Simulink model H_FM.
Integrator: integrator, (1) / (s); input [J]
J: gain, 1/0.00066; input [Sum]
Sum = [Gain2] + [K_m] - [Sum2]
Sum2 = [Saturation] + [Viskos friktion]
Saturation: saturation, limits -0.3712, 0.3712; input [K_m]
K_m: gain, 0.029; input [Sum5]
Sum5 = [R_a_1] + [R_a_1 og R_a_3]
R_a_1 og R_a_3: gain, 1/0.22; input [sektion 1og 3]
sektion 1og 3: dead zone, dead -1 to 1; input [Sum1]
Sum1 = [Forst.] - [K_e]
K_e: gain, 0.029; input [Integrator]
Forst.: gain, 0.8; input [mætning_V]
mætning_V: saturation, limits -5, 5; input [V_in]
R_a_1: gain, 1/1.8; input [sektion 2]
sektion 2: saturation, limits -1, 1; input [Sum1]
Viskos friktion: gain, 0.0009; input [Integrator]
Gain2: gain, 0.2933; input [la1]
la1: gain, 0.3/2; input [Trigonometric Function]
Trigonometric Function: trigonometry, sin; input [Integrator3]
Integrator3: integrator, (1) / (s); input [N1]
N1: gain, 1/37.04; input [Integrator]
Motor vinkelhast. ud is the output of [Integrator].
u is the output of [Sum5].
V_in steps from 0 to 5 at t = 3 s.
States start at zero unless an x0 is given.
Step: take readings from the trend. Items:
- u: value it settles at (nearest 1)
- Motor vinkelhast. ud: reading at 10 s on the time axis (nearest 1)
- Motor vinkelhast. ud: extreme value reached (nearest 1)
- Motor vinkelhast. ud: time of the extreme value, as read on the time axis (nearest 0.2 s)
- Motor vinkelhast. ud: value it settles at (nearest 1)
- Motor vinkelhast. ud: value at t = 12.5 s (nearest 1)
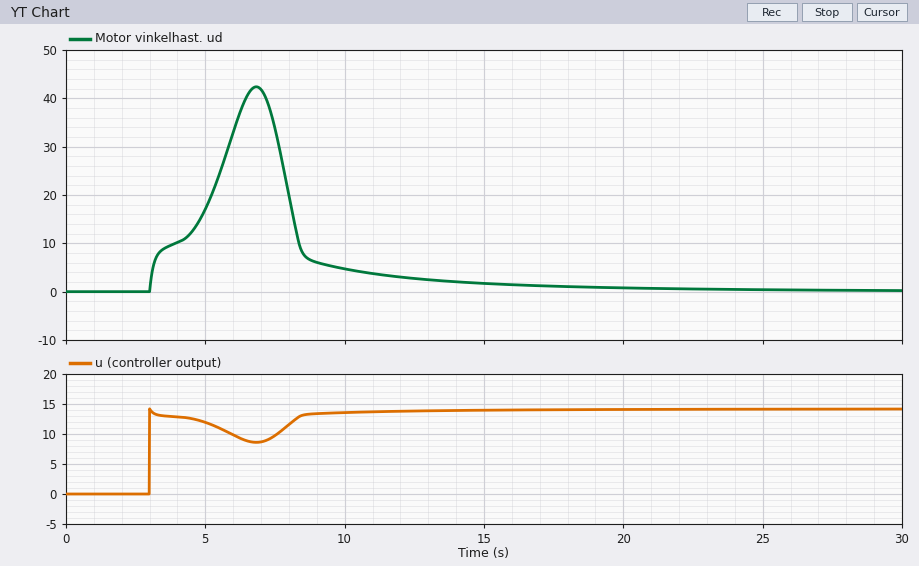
14
5
42
6.8 s
0
3
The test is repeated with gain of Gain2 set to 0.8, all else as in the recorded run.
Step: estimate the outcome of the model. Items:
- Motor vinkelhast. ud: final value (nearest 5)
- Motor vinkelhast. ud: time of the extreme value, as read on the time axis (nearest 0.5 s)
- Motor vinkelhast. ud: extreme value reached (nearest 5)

0
5.5 s
95
